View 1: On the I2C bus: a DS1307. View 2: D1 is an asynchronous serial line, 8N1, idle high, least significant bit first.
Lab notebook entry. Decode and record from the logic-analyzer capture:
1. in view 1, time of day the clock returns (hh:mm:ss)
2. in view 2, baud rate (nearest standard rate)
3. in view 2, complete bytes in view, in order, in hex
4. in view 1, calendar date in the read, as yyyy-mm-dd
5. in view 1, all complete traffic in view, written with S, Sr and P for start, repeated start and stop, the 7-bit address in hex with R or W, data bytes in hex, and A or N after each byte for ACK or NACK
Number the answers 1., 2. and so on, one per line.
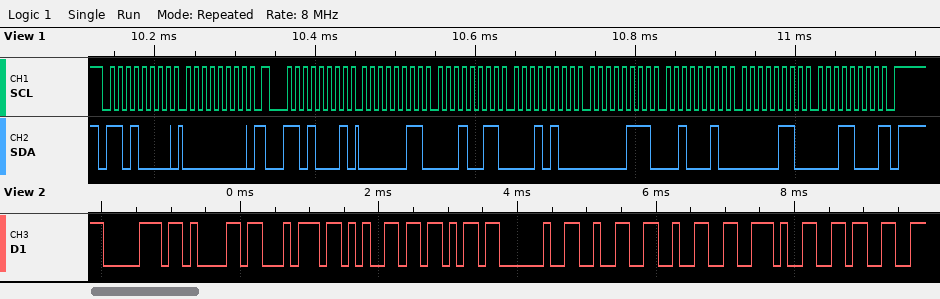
1. 14:13:03
2. 9600 baud
3. 0x70 0x61 0x74 0x65 0x6B 0x20 0x32 0x32 0x2E 0x36
4. 2018-06-22
5. S 68W A 00 A Sr 68R A 03 A 13 A 14 A 07 A 22 A 06 A 18 N P
